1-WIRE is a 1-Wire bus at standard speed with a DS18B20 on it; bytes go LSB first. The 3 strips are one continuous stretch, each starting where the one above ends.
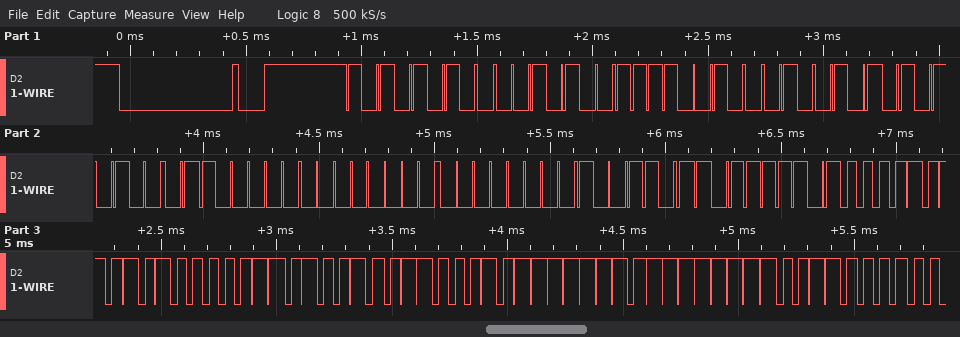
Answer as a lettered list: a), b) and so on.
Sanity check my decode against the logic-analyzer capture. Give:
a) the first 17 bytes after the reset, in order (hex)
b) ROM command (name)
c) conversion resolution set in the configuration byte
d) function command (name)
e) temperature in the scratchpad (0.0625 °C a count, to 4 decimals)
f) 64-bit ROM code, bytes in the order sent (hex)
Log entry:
a) 55 28 4F A4 2A 06 00 00 D9 BE 50 05 4B 46 7F FF 0C
b) Match ROM
c) 12 bits
d) Read Scratchpad
e) 85.0000 °C
f) 28 4F A4 2A 06 00 00 D9
